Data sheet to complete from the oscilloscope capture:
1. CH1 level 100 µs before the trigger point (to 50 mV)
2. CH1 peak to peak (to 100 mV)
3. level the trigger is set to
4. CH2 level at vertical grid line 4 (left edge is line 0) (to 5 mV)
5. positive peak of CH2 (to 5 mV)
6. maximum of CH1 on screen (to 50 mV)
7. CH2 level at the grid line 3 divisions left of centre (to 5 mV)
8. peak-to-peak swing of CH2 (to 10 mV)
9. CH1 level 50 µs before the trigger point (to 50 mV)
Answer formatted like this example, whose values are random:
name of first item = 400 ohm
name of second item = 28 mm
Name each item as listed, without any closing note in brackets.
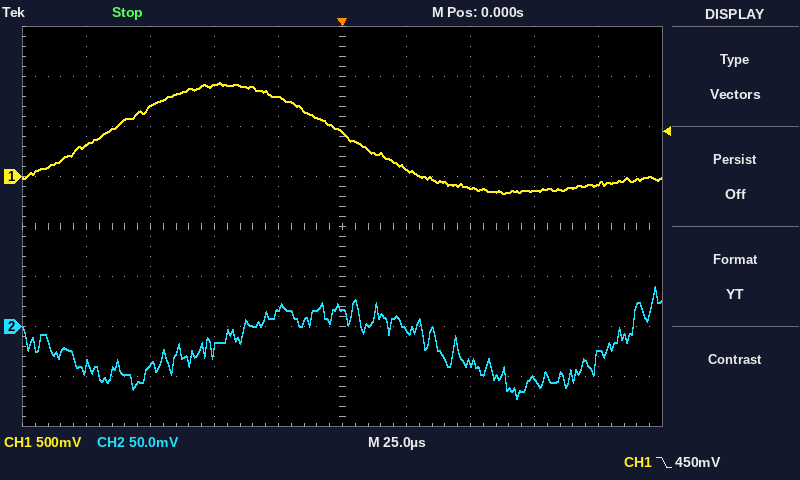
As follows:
CH1 level 100 µs before the trigger point = 300 mV
CH1 peak to peak = 1.10 V
level the trigger is set to = 450 mV
CH2 level at vertical grid line 4 (left edge is line 0) = 15 mV
positive peak of CH2 = 40 mV
maximum of CH1 on screen = 950 mV
CH2 level at the grid line 3 divisions left of centre = -40 mV
peak-to-peak swing of CH2 = 110 mV
CH1 level 50 µs before the trigger point = 900 mV
